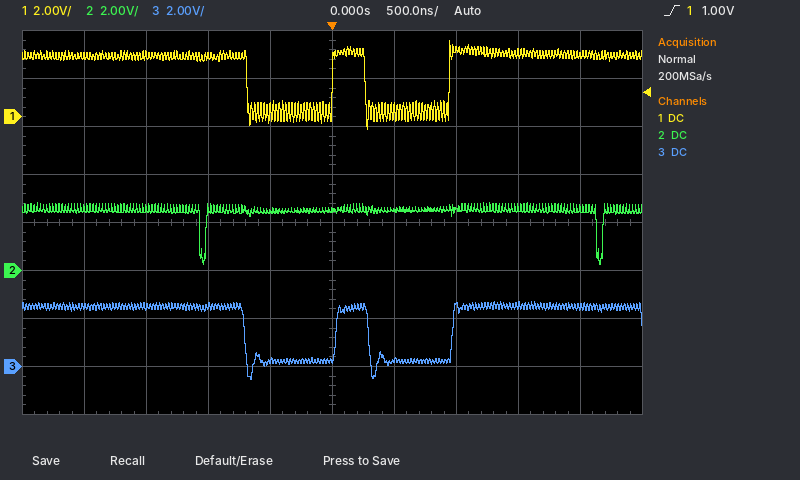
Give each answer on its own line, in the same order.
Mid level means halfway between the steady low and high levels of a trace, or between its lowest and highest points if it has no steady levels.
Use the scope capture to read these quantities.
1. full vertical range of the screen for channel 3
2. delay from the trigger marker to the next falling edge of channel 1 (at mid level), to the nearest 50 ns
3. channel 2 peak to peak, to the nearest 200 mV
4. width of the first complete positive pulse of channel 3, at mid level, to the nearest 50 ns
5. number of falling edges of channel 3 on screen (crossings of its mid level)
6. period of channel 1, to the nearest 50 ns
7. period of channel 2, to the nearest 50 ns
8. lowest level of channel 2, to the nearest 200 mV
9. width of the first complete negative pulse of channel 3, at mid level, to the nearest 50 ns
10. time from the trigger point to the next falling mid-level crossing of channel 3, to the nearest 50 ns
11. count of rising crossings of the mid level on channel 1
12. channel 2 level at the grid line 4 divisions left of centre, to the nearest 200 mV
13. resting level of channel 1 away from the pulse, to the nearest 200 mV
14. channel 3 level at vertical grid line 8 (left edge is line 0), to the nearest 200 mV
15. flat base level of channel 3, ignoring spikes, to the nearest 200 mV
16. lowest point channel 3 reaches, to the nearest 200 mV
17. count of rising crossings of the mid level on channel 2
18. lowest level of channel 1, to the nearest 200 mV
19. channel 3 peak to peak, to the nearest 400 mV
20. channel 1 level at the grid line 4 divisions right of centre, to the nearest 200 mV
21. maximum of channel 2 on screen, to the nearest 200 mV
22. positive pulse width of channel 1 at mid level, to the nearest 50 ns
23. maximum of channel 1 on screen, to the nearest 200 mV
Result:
16 V
250 ns
2.6 V
250 ns
2
950 ns
3.20 µs
200 mV
750 ns
300 ns
2
2.6 V
2.6 V
2.6 V
200 mV
-600 mV
2
-600 mV
3.2 V
2.6 V
2.8 V
250 ns
3.2 V
